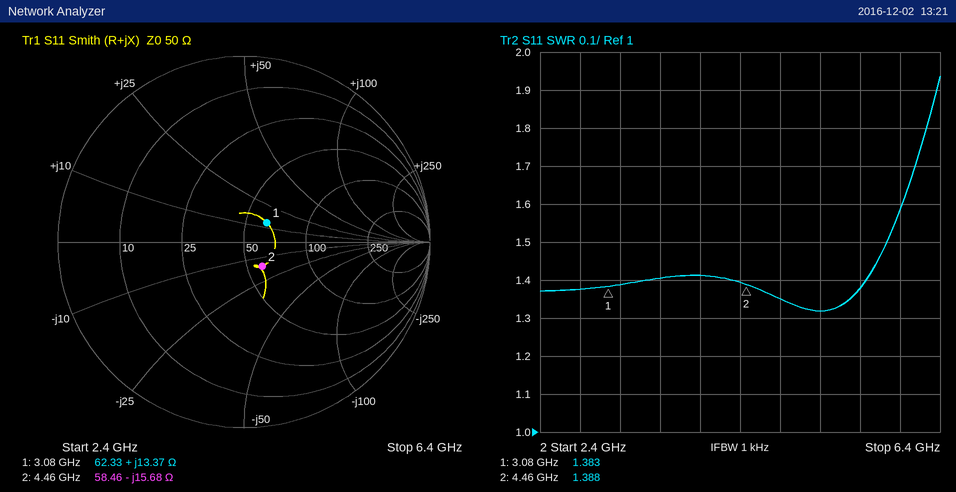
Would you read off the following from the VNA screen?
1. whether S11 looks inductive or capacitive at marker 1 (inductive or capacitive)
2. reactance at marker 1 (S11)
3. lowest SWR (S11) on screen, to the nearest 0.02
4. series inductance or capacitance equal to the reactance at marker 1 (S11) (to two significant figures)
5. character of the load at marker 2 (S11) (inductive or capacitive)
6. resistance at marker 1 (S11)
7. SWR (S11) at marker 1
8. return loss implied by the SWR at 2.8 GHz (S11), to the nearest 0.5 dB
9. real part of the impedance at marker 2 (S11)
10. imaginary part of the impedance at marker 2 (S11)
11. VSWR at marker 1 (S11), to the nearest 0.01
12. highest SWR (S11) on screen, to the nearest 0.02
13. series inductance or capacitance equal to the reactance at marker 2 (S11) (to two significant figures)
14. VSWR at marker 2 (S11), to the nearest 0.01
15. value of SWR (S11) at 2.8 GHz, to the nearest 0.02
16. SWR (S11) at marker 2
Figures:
inductive
+13.37 Ω
1.32
690 pH
capacitive
62.33 Ω
1.383
16.0 dB
58.46 Ω
-15.68 Ω
1.38
1.94
2.3 pF
1.39
1.38
1.388
